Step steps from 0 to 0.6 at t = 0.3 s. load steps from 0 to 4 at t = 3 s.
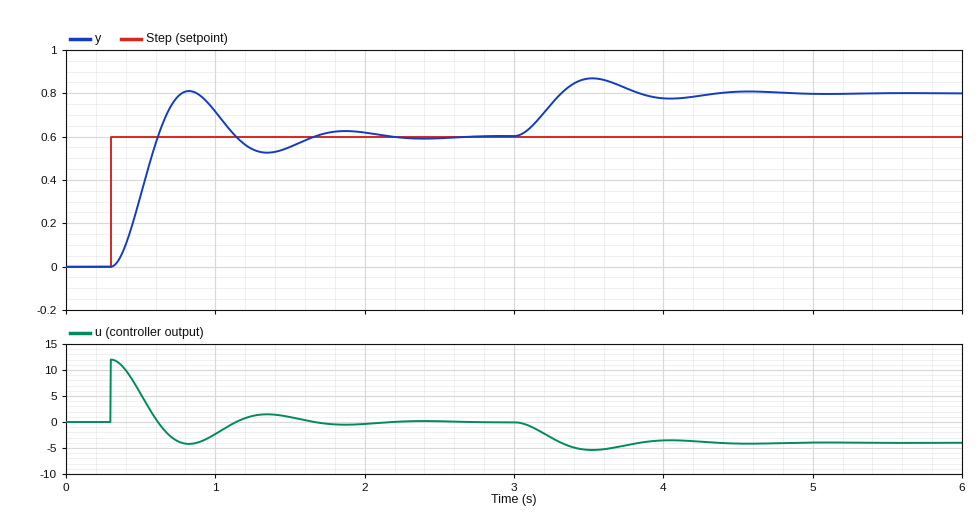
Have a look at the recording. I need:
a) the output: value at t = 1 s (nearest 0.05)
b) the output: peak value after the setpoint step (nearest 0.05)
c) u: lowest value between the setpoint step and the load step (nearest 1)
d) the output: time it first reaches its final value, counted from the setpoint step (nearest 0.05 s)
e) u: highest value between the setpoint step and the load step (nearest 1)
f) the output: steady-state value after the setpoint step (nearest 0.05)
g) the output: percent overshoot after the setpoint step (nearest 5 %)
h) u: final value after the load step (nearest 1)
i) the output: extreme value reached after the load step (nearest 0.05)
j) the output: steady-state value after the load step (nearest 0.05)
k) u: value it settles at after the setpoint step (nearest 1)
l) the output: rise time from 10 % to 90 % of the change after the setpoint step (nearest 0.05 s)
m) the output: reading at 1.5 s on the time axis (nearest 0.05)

0.70
0.80
-4
0.30 s
12
0.60
35 %
-4
0.85
0.80
0
0.20 s
0.55
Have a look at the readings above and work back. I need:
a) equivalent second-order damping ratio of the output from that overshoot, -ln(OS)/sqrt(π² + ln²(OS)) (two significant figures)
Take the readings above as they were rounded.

0.32
